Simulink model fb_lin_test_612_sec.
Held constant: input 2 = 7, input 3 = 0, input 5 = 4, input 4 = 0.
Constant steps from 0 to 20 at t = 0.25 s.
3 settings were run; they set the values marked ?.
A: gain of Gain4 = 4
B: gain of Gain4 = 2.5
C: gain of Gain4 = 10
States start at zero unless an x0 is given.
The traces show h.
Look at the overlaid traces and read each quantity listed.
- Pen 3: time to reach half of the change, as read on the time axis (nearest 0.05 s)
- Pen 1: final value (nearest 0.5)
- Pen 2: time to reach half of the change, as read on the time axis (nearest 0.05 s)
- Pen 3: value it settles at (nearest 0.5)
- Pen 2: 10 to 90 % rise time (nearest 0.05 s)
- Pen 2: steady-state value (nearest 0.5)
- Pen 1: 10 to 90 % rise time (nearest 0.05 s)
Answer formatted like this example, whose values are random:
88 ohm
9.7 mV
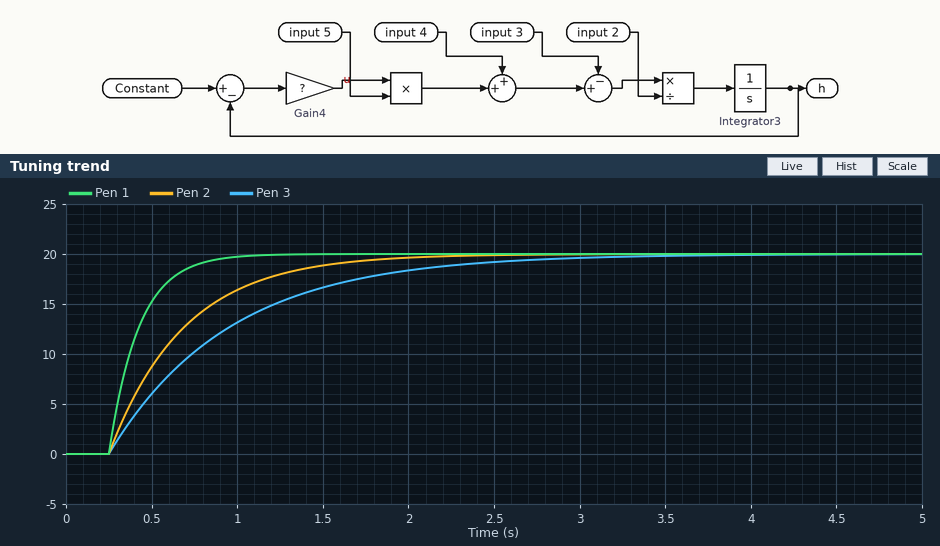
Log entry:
0.75 s
20.0
0.55 s
20.0
0.95 s
20.0
0.40 s
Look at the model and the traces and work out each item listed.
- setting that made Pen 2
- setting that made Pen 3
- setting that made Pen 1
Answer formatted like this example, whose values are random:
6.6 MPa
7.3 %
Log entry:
A
B
C
